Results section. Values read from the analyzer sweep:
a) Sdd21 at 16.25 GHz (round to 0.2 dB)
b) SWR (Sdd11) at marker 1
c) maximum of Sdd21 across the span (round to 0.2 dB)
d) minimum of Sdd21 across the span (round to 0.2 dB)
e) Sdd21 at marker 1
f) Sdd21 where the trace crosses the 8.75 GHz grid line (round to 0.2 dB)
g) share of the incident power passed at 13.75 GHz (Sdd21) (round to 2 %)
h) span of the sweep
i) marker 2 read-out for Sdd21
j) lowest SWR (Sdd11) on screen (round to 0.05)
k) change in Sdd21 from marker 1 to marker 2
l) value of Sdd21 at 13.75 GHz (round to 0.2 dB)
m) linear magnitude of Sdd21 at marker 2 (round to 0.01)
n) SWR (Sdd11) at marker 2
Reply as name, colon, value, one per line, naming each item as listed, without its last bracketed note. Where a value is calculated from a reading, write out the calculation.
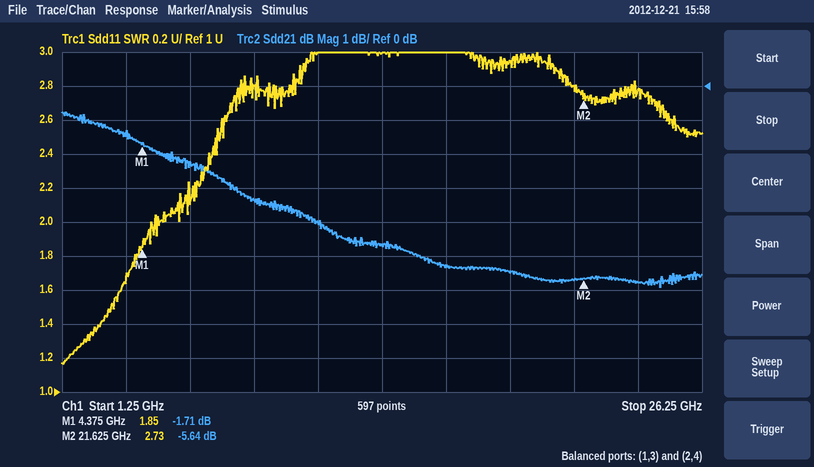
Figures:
Sdd21 at 16.25 GHz: -5.2 dB
SWR (Sdd11) at marker 1: 1.85
maximum of Sdd21 across the span: -0.8 dB
minimum of Sdd21 across the span: -6.0 dB
Sdd21 at marker 1: -1.71 dB
Sdd21 where the trace crosses the 8.75 GHz grid line: -3.4 dB
share of the incident power passed at 13.75 GHz (Sdd21): 10^(-4.6/10) ≈ 34.7 %, so 34 % to the nearest 2 %
span of the sweep: 25 GHz
marker 2 read-out for Sdd21: -5.64 dB
lowest SWR (Sdd11) on screen: 1.15
change in Sdd21 from marker 1 to marker 2: -5.64 − (-1.71) = -3.93 dB
value of Sdd21 at 13.75 GHz: -4.6 dB
linear magnitude of Sdd21 at marker 2: 10^(-5.64/20) ≈ 0.52
SWR (Sdd11) at marker 2: 2.73
